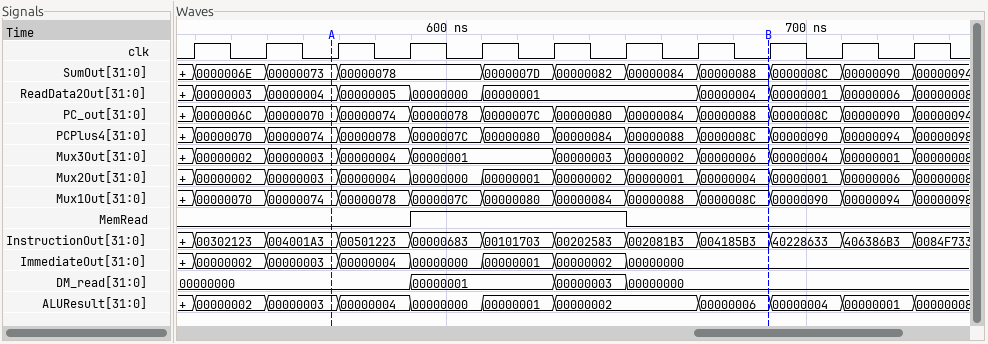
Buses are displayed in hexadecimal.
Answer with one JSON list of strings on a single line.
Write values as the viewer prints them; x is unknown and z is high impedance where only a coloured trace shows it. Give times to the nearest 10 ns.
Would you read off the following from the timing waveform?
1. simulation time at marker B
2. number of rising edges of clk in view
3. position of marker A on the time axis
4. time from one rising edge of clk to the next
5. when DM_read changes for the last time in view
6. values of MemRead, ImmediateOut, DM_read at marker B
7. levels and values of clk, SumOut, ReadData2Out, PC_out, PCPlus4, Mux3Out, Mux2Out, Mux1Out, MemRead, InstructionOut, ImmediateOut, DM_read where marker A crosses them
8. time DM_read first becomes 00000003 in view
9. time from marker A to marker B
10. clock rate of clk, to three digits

["690 ns", "11", "570 ns", "20 ns", "650 ns", "MemRead=0, ImmediateOut=00000000, DM_read=00000000", "clk=0, SumOut=00000073, ReadData2Out=00000004, PC_out=00000070, PCPlus4=00000074, Mux3Out=00000003, Mux2Out=00000003, Mux1Out=00000074, MemRead=0, InstructionOut=004001A3, ImmediateOut=00000003, DM_read=00000000", "630 ns", "120 ns", "50.0 MHz"]
